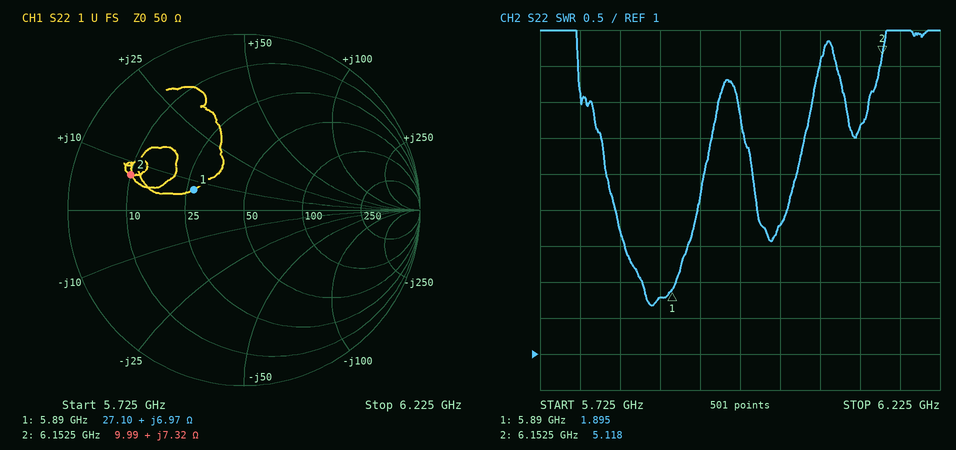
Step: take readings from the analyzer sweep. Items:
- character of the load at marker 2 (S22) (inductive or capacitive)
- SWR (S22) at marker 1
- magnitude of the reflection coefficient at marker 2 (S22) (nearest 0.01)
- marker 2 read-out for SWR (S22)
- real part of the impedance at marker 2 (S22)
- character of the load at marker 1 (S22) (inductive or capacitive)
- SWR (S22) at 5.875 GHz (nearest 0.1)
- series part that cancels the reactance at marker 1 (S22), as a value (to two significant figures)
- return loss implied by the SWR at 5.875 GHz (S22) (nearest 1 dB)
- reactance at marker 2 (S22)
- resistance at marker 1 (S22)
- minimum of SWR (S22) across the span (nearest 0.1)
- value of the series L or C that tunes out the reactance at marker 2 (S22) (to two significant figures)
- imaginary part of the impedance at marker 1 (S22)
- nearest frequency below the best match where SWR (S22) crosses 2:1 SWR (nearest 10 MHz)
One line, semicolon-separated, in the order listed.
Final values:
inductive; 1.895; 0.67; 5.118; 9.99 Ω; inductive; 1.8; 3.9 pF; 11 dB; +7.32 Ω; 27.10 Ω; 1.7; 3.5 pF; +6.97 Ω; 5.85 GHz
